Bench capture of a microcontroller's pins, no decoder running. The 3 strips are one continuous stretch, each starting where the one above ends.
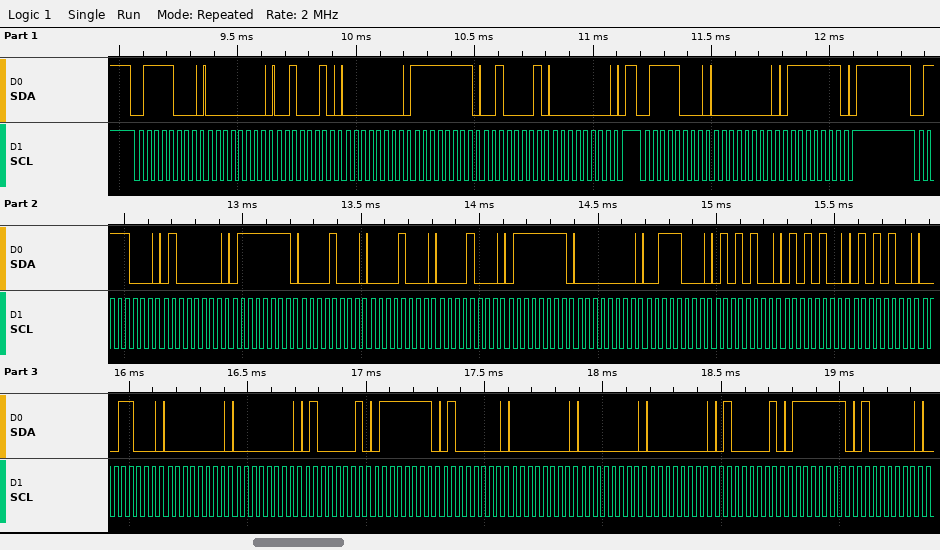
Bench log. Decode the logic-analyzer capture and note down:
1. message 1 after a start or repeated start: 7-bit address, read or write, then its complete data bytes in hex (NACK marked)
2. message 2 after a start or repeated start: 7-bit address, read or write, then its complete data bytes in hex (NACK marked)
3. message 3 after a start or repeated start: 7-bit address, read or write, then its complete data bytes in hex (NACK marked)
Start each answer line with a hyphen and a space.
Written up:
- 0x3C write: 00 22 00 FF 21 00
- 0x3C write: 00 7F
- 0x3C write: 40 7F 08 08 08 7F 00 38 54 54 54 18 00 00 41 7F 40 00 00 00 41 7F 40
